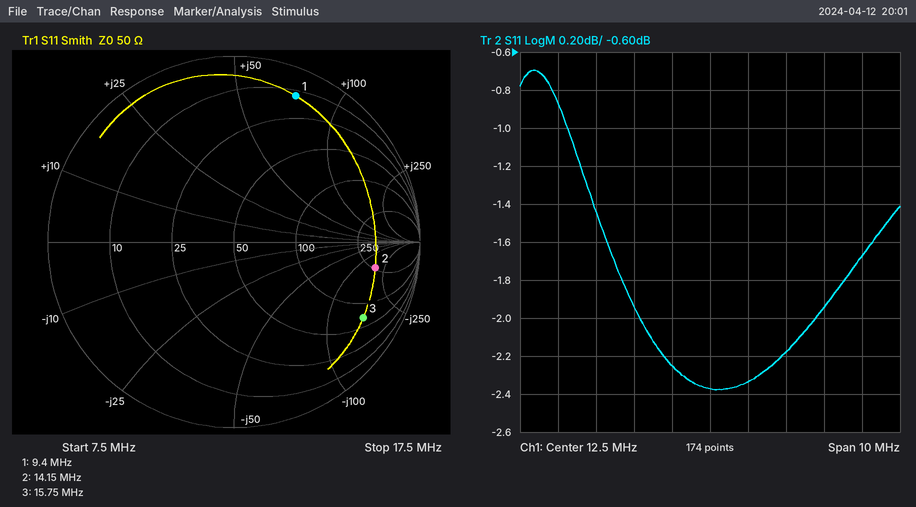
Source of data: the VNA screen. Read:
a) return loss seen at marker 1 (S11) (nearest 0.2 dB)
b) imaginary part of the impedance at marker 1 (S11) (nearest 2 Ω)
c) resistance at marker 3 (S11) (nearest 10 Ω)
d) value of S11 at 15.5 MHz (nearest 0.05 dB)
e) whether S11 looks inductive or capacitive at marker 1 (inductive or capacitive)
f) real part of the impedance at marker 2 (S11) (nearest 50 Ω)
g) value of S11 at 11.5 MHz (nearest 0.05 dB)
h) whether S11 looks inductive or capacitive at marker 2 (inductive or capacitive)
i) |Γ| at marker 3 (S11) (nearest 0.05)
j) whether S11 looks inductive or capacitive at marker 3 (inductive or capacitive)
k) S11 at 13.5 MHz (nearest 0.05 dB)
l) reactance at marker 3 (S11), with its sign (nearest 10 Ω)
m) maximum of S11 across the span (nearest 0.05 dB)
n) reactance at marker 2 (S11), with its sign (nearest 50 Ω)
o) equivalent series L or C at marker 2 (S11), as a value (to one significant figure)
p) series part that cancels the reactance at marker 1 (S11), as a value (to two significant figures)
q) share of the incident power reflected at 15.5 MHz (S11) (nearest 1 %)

1.4 dB
+74 Ω
70 Ω
-1.95 dB
inductive
250 Ω
-2.25 dB
capacitive
0.80
capacitive
-2.35 dB
-160 Ω
-0.70 dB
-200 Ω
60 pF
230 pF
64 %
